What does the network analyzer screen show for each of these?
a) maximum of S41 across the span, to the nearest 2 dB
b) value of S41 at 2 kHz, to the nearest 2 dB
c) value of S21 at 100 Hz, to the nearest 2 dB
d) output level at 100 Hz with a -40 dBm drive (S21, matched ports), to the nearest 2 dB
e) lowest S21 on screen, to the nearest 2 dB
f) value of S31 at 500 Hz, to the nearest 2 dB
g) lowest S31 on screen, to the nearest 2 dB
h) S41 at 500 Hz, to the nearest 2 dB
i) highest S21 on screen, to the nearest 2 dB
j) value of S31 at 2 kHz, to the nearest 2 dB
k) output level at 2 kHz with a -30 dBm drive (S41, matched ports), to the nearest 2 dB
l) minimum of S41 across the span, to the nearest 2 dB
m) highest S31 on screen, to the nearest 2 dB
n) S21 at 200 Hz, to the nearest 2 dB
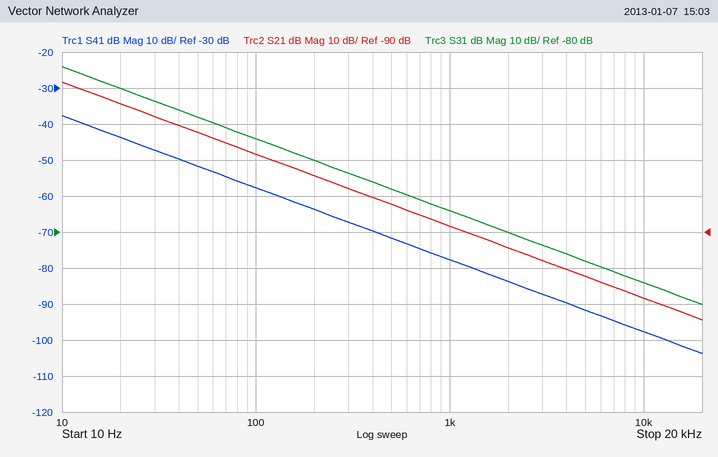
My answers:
-38 dB
-84 dB
-68 dB
-108 dBm
-114 dB
-68 dB
-100 dB
-72 dB
-48 dB
-80 dB
-114 dBm
-104 dB
-34 dB
-74 dB
